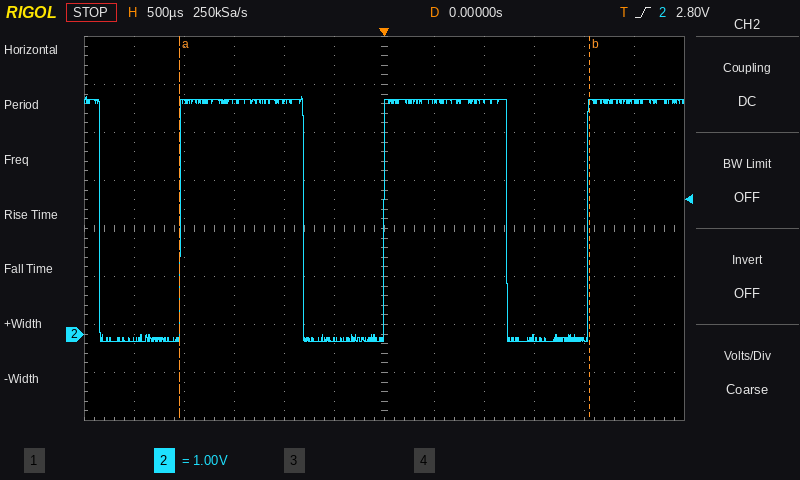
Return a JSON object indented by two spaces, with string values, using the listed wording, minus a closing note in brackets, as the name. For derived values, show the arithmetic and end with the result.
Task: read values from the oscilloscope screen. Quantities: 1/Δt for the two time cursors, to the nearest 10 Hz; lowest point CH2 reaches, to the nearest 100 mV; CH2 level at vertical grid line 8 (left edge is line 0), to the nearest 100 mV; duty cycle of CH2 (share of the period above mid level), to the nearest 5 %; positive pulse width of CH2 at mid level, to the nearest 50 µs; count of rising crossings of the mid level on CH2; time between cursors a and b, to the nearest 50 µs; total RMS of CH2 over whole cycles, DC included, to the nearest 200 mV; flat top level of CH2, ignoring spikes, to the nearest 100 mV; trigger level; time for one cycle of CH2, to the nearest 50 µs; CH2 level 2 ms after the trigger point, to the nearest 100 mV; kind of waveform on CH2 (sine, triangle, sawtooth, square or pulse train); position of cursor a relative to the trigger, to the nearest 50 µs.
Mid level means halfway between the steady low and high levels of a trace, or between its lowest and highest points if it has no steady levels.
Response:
{
  "1/Δt for the two time cursors, to the nearest 10 Hz": "1 / 4.10 ms ≈ 240 Hz",
  "lowest point CH2 reaches, to the nearest 100 mV": "-200 mV",
  "CH2 level at vertical grid line 8 (left edge is line 0), to the nearest 100 mV": "4.8 V",
  "duty cycle of CH2 (share of the period above mid level), to the nearest 5 %": "1.25 ms / 2.05 ms ≈ 61.0 %, so 60 % to the nearest 5 %",
  "positive pulse width of CH2 at mid level, to the nearest 50 µs": "1.25 ms",
  "count of rising crossings of the mid level on CH2": "3",
  "time between cursors a and b, to the nearest 50 µs": "4.10 ms",
  "total RMS of CH2 over whole cycles, DC included, to the nearest 200 mV": "√(0.6 × (4.9 V)² + 0.4 × (-200 mV)²) ≈ 3.8 V",
  "flat top level of CH2, ignoring spikes, to the nearest 100 mV": "4.9 V",
  "trigger level": "2.80 V",
  "time for one cycle of CH2, to the nearest 50 µs": "2.05 ms",
  "CH2 level 2 ms after the trigger point, to the nearest 100 mV": "-100 mV",
  "kind of waveform on CH2": "pulse train",
  "position of cursor a relative to the trigger, to the nearest 50 µs": "-2.05 ms"
}
